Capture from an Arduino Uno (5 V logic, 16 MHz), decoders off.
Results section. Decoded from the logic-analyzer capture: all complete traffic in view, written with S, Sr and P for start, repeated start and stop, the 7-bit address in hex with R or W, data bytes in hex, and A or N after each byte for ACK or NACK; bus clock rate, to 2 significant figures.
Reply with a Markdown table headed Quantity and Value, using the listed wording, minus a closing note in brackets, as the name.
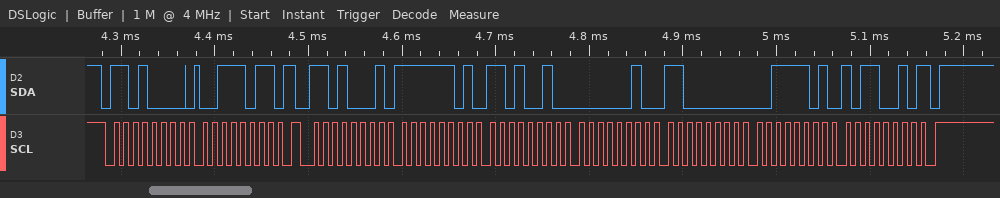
| Quantity | Value |
|---|---|
| all complete traffic in view, written with S, Sr and P for start, repeated start and stop, the 7-bit address in hex with R or W, data bytes in hex, and A or N after each byte for ACK or NACK | S 68W A 3B A Sr 68R A FD A D2 A 02 A C0 A 3D A B2 N P |
| bus clock rate, to 2 significant figures | 100 kHz |
